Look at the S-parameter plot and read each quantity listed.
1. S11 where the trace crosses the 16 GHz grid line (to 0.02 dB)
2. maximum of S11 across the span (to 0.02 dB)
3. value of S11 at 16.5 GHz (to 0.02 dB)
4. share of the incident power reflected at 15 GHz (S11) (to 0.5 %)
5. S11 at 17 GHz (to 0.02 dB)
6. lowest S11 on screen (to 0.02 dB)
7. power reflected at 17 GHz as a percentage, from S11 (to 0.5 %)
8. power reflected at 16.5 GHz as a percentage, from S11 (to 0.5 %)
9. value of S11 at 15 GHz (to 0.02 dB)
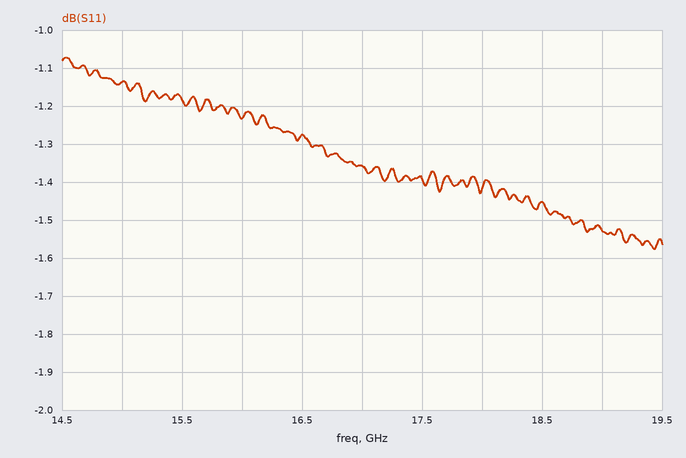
-1.24 dB
-1.08 dB
-1.28 dB
77.0 %
-1.36 dB
-1.58 dB
73.0 %
74.5 %
-1.14 dB
